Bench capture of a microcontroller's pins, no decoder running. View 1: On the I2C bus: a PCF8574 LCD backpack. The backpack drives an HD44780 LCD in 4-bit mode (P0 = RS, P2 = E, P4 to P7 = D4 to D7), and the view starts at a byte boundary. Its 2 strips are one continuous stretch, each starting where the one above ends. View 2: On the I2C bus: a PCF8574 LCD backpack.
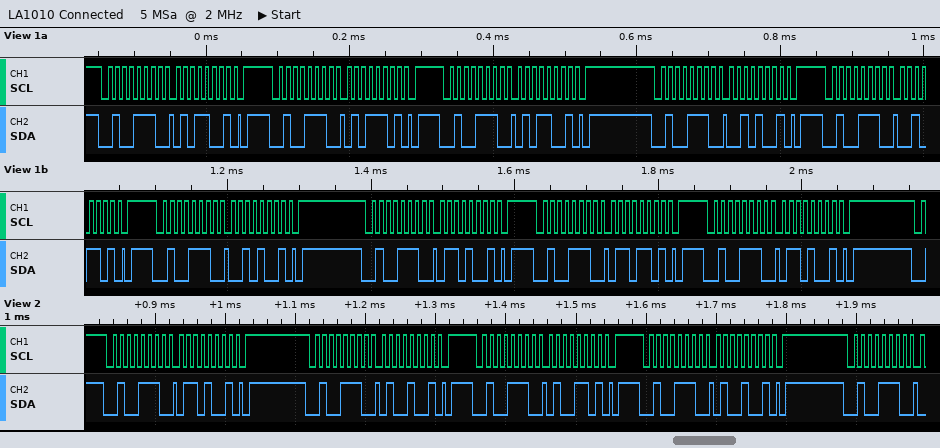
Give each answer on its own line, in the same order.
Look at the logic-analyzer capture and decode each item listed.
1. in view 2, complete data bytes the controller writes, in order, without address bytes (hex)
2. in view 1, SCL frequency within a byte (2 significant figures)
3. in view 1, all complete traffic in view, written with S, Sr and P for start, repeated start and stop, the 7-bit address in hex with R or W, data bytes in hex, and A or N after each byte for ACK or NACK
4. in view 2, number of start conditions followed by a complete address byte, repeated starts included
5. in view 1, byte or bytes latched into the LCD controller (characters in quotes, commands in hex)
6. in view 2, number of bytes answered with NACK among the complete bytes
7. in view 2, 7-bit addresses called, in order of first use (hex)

69 49 4D 49
100 kHz
S 27W A 59 A P S 27W A 5D A P S 27W A 59 A P S 27W A 29 A P S 27W A 2D A P S 27W A 29 A P S 27W A 69 A P S 27W A 6D A P S 27W A 69 A P
5
'R'
0
0x27
